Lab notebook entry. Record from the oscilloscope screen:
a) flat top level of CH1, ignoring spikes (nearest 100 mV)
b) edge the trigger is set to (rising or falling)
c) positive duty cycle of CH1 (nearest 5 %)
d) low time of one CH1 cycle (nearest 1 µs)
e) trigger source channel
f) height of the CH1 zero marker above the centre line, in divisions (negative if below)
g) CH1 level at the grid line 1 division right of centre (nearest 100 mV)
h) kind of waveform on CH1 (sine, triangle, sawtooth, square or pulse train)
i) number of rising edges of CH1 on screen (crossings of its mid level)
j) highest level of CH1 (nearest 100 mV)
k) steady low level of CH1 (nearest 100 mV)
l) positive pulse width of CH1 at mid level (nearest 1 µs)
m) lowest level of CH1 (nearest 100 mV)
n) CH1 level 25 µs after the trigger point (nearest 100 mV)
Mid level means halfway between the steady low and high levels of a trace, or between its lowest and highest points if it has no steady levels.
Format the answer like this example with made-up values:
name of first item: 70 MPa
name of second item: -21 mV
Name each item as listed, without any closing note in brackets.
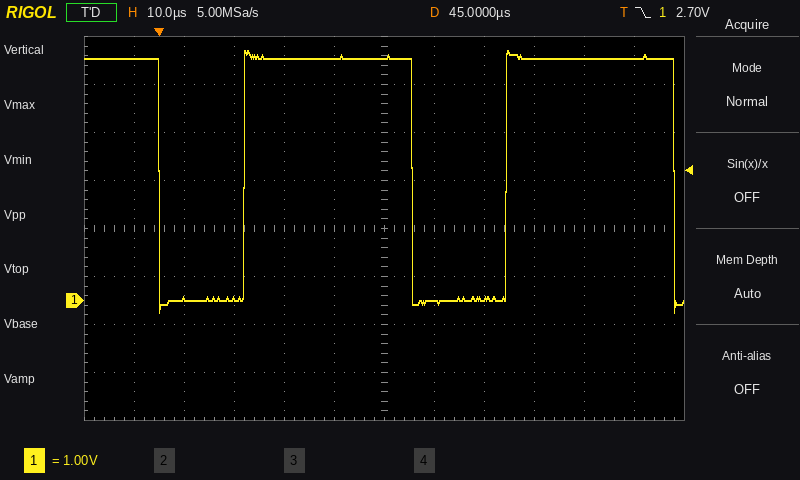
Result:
flat top level of CH1, ignoring spikes: 5.0 V
edge the trigger is set to: falling
positive duty cycle of CH1: 65 %
low time of one CH1 cycle: 18 µs
trigger source channel: CH1
height of the CH1 zero marker above the centre line, in divisions: -1.5 div
CH1 level at the grid line 1 division right of centre: 0.0 V
kind of waveform on CH1: pulse train
number of rising edges of CH1 on screen: 2
highest level of CH1: 5.2 V
steady low level of CH1: 0.0 V
positive pulse width of CH1 at mid level: 34 µs
lowest level of CH1: -200 mV
CH1 level 25 µs after the trigger point: 5.0 V
